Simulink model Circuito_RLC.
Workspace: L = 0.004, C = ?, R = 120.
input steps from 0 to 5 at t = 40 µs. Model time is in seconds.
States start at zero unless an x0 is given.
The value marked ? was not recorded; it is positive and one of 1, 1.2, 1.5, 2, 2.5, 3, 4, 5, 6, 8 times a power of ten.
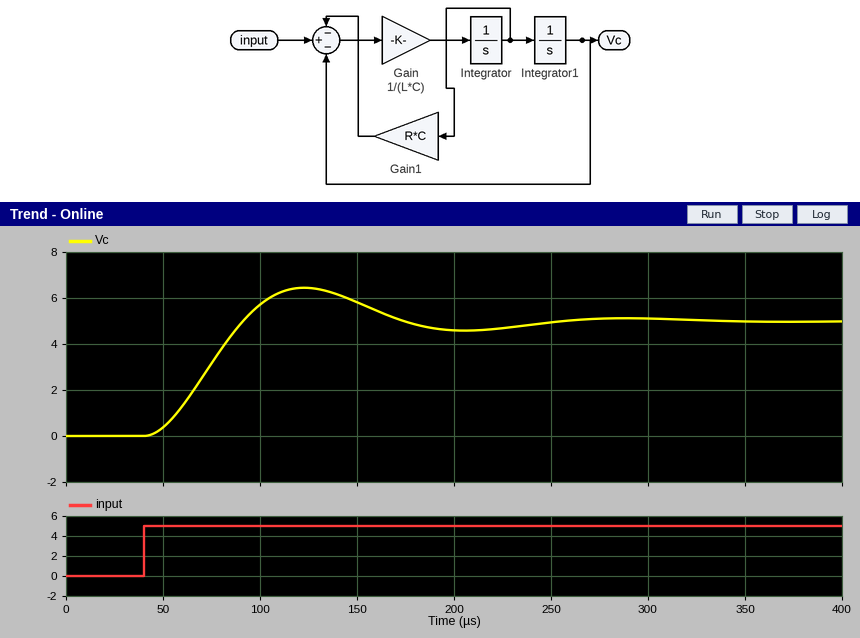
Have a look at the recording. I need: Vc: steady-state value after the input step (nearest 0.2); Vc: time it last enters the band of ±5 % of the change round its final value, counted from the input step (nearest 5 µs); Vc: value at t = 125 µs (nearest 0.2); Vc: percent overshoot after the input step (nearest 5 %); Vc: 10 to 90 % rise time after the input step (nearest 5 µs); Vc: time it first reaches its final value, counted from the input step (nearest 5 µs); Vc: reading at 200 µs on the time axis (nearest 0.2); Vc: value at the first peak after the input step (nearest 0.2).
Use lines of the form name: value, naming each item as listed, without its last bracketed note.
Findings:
Vc: steady-state value after the input step: 5.0
Vc: time it last enters the band of ±5 % of the change round its final value, counted from the input step: 190 µs
Vc: value at t = 125 µs: 6.4
Vc: percent overshoot after the input step: 30 %
Vc: 10 to 90 % rise time after the input step: 35 µs
Vc: time it first reaches its final value, counted from the input step: 50 µs
Vc: reading at 200 µs on the time axis: 4.6
Vc: value at the first peak after the input step: 6.4
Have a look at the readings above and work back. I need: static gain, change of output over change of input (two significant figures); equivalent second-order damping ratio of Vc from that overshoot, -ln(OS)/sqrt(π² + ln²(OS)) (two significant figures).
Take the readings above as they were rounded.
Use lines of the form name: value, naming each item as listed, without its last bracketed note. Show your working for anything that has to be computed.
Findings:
static gain, change of output over change of input: (5 - 0) / (5 - 0) = 1.0
equivalent second-order damping ratio of Vc from that overshoot, -ln(OS)/sqrt(π² + ln²(OS)): ln(0.3) = -1.204; 1.204 / sqrt(9.870 + 1.450) = 0.36
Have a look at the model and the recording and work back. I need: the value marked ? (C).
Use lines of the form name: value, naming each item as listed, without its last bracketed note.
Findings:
the value marked ?: 1.5e-07
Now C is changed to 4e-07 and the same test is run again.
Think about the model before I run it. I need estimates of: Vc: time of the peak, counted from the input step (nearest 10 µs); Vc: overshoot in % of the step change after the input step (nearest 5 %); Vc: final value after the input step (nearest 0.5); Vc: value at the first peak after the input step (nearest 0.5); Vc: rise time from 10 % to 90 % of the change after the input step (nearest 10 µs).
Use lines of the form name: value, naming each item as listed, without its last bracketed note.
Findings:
Vc: time of the peak, counted from the input step: 160 µs
Vc: overshoot in % of the step change after the input step: 10 %
Vc: final value after the input step: 5.0
Vc: value at the first peak after the input step: 5.5
Vc: rise time from 10 % to 90 % of the change after the input step: 70 µs
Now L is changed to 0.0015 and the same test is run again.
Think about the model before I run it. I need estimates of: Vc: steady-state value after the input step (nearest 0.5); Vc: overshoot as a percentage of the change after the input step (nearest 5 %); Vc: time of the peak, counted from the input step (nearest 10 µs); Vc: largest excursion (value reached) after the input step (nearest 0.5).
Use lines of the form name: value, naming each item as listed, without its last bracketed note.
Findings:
Vc: steady-state value after the input step: 5.0
Vc: overshoot as a percentage of the change after the input step: 10 %
Vc: time of the peak, counted from the input step: 60 µs
Vc: largest excursion (value reached) after the input step: 5.5
